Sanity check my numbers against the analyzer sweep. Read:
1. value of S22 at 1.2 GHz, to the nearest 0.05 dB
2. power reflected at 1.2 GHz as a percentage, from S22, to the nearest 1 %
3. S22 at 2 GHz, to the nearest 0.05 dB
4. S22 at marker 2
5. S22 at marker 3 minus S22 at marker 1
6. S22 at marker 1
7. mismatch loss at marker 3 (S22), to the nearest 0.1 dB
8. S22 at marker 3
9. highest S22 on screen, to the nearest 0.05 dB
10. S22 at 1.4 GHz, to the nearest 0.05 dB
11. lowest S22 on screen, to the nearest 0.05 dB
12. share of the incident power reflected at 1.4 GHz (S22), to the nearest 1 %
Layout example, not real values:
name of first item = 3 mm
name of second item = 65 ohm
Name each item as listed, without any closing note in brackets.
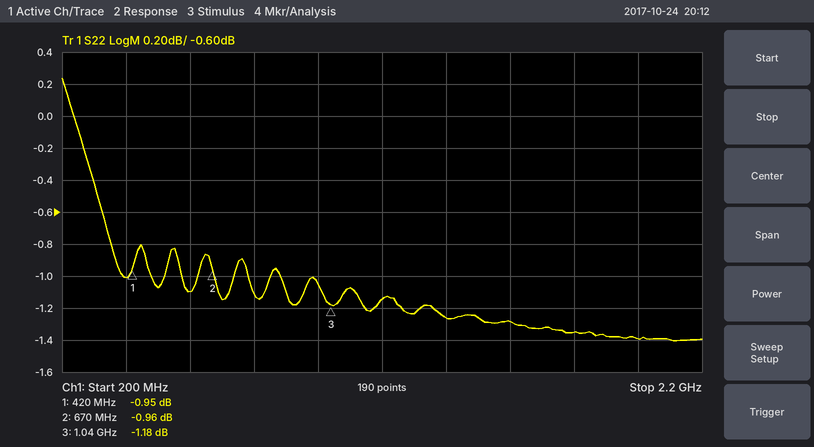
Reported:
value of S22 at 1.2 GHz, to the nearest 0.05 dB = -1.15 dB
power reflected at 1.2 GHz as a percentage, from S22, to the nearest 1 % = 77 %
S22 at 2 GHz, to the nearest 0.05 dB = -1.40 dB
S22 at marker 2 = -0.96 dB
S22 at marker 3 minus S22 at marker 1 = -0.23 dB
S22 at marker 1 = -0.95 dB
mismatch loss at marker 3 (S22), to the nearest 0.1 dB = 6.2 dB
S22 at marker 3 = -1.18 dB
highest S22 on screen, to the nearest 0.05 dB = 0.25 dB
S22 at 1.4 GHz, to the nearest 0.05 dB = -1.25 dB
lowest S22 on screen, to the nearest 0.05 dB = -1.40 dB
share of the incident power reflected at 1.4 GHz (S22), to the nearest 1 % = 75 %
